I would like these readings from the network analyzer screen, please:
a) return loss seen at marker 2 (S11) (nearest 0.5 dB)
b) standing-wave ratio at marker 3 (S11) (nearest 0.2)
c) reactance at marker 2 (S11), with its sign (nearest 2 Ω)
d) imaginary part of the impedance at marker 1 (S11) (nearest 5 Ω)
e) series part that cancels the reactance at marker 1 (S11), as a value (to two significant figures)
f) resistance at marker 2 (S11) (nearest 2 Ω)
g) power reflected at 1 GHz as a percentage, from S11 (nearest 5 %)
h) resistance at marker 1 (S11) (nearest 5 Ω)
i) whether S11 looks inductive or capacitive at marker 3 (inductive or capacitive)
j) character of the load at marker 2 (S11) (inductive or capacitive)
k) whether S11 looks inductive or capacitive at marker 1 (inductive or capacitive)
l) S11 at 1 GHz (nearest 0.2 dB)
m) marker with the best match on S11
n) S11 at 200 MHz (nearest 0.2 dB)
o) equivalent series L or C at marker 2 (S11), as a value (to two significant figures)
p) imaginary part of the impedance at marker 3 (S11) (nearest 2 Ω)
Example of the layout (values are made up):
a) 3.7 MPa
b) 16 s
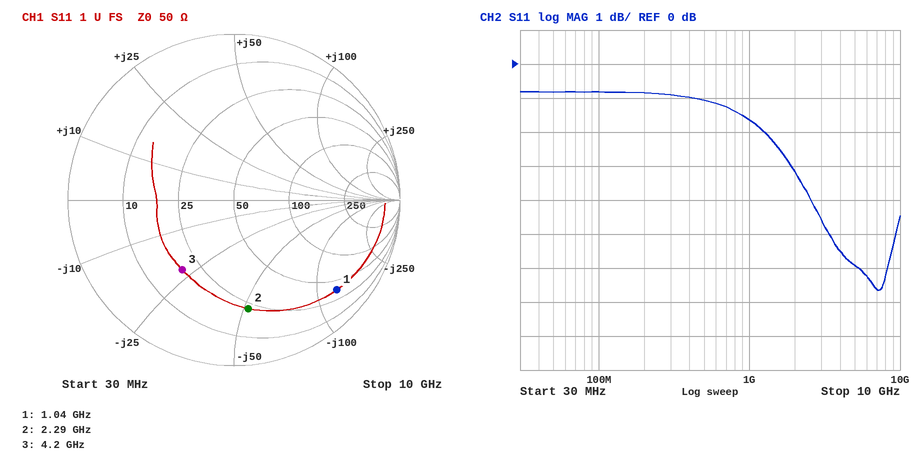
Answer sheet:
a) 3.5 dB
b) 3.2
c) -52 Ω
d) -125 Ω
e) 19 nH
f) 22 Ω
g) 70 %
h) 35 Ω
i) capacitive
j) capacitive
k) capacitive
l) -1.6 dB
m) marker 3
n) -0.8 dB
o) 1.3 pF
p) -22 Ω
